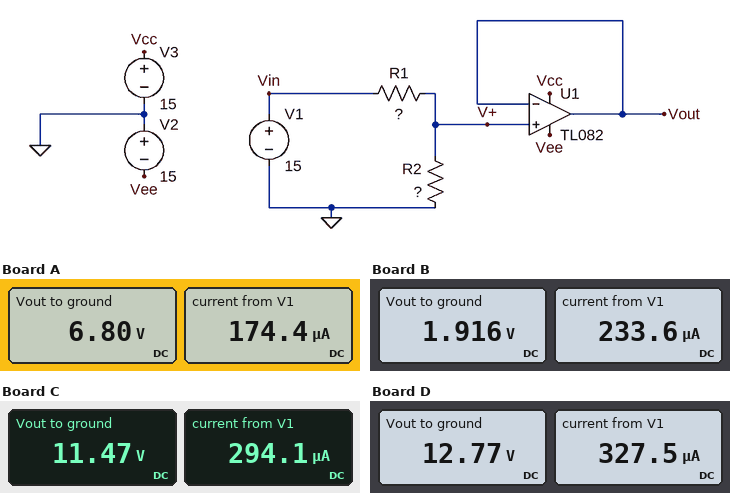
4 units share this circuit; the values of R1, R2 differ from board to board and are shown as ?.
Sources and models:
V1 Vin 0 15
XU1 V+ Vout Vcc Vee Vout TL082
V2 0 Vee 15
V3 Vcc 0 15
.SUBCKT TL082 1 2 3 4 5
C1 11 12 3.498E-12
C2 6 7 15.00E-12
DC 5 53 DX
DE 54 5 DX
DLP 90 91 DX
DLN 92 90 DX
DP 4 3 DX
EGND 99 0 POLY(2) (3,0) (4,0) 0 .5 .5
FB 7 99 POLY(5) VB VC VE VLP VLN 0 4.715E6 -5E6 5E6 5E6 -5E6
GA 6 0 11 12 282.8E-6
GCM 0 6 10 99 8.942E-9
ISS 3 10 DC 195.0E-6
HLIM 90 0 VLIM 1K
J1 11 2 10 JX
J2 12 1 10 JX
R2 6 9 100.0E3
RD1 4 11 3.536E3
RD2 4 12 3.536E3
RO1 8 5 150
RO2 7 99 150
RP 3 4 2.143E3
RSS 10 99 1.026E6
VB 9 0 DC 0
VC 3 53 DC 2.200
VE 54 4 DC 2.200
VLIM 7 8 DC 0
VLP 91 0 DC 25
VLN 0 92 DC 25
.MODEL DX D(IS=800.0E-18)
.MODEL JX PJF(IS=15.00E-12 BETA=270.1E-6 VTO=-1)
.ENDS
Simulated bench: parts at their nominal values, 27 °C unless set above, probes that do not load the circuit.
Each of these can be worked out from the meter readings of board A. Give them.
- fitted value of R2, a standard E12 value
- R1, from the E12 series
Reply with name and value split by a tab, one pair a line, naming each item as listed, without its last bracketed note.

fitted value of R2, a standard E12 value	39 kΩ
R1, from the E12 series	47 kΩ
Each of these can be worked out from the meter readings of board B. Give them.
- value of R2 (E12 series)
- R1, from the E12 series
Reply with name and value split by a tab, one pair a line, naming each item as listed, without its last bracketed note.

value of R2	8.2 kΩ
R1, from the E12 series	56 kΩ
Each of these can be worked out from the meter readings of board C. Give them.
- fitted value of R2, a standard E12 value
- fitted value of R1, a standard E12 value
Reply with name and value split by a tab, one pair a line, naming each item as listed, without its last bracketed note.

fitted value of R2, a standard E12 value	39 kΩ
fitted value of R1, a standard E12 value	12 kΩ
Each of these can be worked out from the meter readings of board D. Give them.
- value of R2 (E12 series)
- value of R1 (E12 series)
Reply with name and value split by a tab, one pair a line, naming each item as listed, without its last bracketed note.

value of R2	39 kΩ
value of R1	6.8 kΩ
